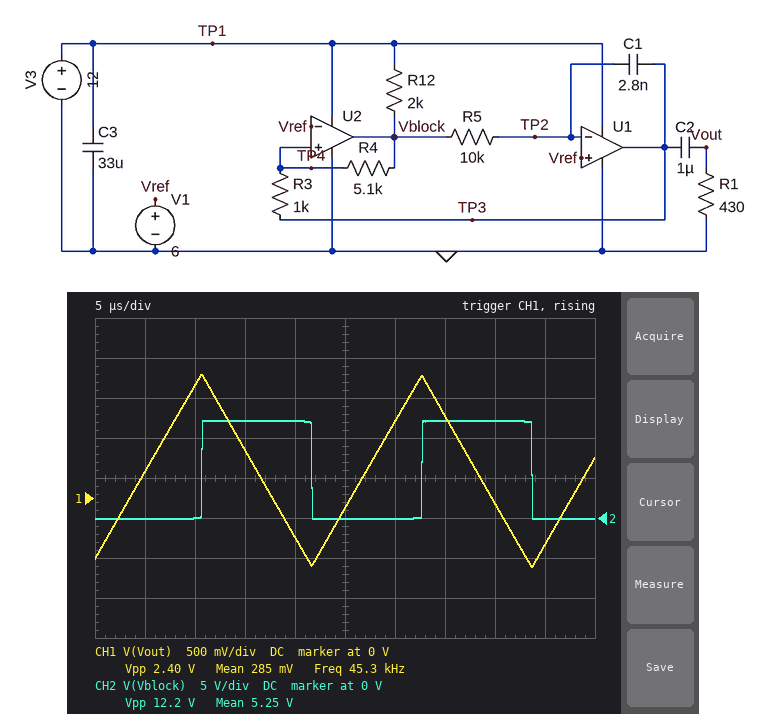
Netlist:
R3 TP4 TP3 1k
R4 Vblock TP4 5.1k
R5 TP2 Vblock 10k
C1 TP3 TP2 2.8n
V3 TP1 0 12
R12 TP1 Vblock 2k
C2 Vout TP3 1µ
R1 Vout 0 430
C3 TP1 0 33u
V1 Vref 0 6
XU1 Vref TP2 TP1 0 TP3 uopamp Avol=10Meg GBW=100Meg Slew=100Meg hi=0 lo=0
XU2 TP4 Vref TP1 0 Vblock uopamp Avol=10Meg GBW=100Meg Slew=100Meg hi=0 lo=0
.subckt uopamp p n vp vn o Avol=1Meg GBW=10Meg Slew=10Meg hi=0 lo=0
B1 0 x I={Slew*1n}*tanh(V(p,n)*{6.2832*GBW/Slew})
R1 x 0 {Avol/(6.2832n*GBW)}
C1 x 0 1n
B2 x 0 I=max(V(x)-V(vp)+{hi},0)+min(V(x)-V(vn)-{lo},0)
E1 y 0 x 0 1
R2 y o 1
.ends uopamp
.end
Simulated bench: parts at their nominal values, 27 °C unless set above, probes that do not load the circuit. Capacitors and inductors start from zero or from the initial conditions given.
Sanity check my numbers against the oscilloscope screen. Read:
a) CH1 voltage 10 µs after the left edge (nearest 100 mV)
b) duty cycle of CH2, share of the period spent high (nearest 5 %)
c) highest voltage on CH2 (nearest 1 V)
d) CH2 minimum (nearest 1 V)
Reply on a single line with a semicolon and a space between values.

1.4 V; 50 %; 12 V; 0 V
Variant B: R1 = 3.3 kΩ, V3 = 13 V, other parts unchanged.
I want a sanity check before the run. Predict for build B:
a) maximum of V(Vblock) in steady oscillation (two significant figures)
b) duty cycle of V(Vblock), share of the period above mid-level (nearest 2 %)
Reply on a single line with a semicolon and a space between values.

13 V; 46 %
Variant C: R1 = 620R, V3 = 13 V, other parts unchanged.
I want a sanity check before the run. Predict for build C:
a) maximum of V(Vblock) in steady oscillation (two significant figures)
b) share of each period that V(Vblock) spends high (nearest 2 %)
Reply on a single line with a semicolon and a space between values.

13 V; 46 %
